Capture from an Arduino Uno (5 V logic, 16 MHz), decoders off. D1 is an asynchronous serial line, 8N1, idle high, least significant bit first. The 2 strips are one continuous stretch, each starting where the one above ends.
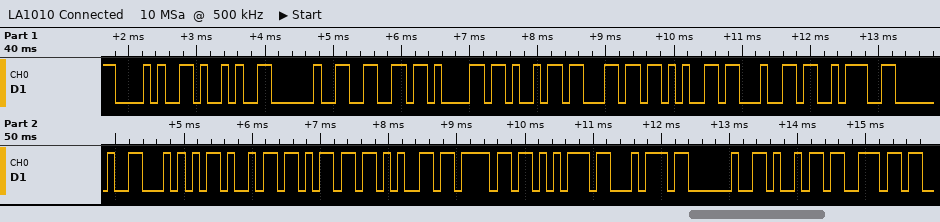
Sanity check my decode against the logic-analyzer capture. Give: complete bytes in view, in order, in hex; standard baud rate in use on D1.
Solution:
0x28 0x29 0x20 0x66 0x61 0x69 0x6C 0x65 0x64 0x3A 0x20 0x54 0x69 0x6D 0x65 0x6F 0x75 0x74 0x20 0x69 0x6E
9600 baud
